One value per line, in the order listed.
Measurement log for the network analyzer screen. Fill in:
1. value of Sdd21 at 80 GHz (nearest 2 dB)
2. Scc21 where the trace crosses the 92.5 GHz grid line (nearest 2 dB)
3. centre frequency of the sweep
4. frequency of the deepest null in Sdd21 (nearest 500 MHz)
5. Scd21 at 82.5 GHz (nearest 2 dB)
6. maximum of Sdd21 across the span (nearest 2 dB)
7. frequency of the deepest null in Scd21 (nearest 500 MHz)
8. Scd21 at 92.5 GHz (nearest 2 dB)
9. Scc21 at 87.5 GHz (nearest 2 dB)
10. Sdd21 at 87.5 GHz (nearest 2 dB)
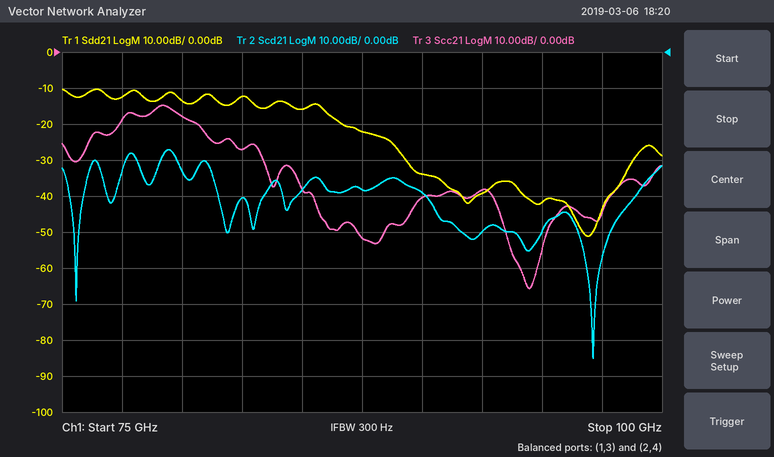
-14 dB
-38 dB
87.5 GHz
97.0 GHz
-40 dB
-10 dB
97.0 GHz
-50 dB
-52 dB
-22 dB
